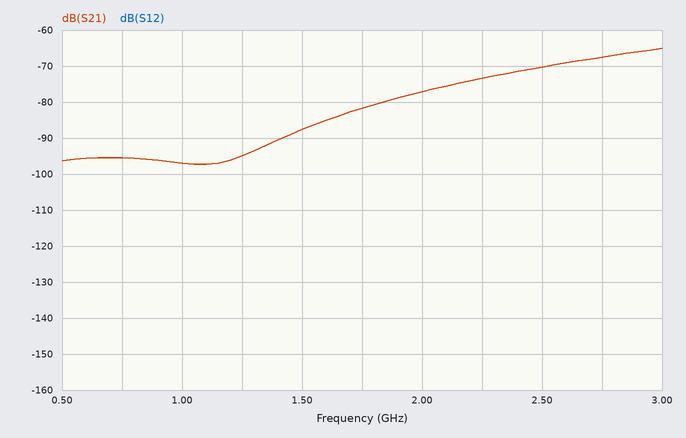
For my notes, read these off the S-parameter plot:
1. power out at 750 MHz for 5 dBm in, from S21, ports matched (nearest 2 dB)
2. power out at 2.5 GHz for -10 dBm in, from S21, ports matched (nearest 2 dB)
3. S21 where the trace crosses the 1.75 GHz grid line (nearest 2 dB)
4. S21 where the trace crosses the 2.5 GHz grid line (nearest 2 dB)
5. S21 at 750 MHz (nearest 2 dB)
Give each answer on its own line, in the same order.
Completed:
-90 dBm
-80 dBm
-82 dB
-70 dB
-96 dB
